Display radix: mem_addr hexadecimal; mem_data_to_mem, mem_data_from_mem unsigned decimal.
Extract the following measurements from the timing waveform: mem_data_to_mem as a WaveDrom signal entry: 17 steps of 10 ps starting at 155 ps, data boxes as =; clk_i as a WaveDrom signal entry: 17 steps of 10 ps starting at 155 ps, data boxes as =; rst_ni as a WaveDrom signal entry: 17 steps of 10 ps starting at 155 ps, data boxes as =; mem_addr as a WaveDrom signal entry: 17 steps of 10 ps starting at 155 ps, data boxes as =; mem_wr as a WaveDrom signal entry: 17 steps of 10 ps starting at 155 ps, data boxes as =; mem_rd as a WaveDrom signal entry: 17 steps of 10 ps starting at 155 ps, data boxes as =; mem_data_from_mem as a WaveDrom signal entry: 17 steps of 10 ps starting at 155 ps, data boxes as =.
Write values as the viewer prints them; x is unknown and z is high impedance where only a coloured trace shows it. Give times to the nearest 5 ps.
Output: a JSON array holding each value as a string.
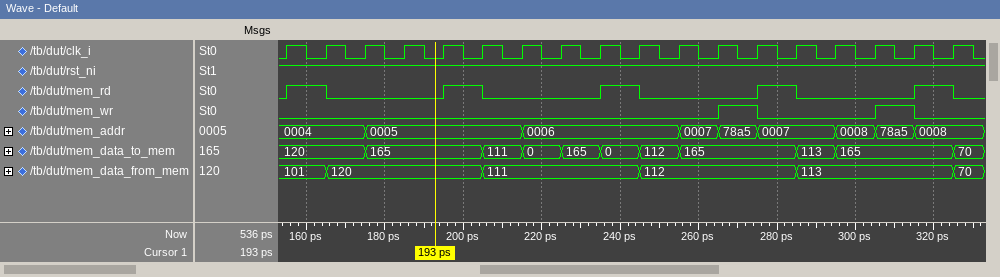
["{name: 'mem_data_to_mem', wave: '=.=..======..==..', data: '120 165 111 0 165 0 112 165 113 165'}", "{name: 'clk_i', wave: 'p................'}", "{name: 'rst_ni', wave: '1................'}", "{name: 'mem_addr', wave: '=.=...=...===.===', data: '0004 0005 0006 0007 78a5 0007 0008 78a5 0008'}", "{name: 'mem_wr', wave: '0..........10..10'}", "{name: 'mem_rd', wave: '10..10..10..10..1'}", "{name: 'mem_data_from_mem', wave: '==...=...=...=...', data: '101 120 111 112 113'}"]
